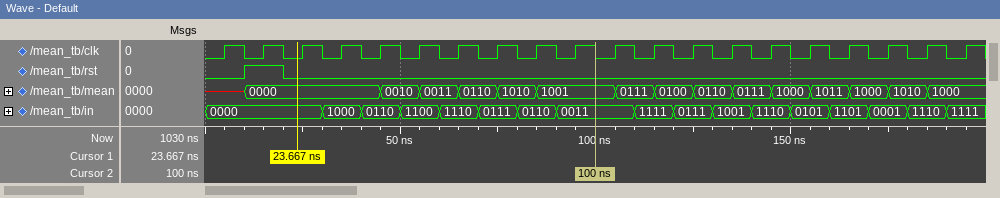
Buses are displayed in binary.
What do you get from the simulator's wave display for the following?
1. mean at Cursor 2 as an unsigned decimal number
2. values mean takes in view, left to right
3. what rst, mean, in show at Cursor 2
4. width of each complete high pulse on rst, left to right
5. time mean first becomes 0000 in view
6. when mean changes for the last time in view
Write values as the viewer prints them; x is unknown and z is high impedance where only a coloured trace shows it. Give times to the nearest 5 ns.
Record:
9
x, 0000, 0010, 0011, 0110, 1010, 1001, 0111, 0100, 0110, 0111, 1000, 1011, 1000, 1010, 1000
rst=0, mean=1001, in=0011
10 ns
10 ns
185 ns
